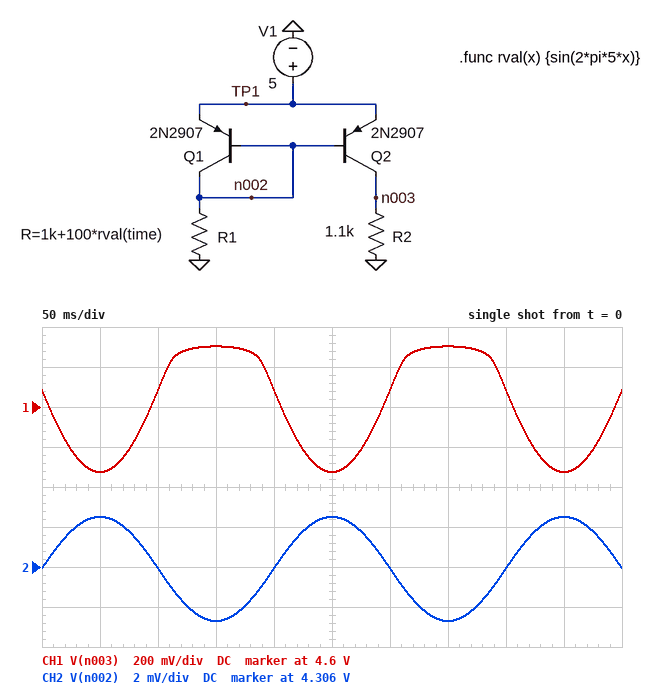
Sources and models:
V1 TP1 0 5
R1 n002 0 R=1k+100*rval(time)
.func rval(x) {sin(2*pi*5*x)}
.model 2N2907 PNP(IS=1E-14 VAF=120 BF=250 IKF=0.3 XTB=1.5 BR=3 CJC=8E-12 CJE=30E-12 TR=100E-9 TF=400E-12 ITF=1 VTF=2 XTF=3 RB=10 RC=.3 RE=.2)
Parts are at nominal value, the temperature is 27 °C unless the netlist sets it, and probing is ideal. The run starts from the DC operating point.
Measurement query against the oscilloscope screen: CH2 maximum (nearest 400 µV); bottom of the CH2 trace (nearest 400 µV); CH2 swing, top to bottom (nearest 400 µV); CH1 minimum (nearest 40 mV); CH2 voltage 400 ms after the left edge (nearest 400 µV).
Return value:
4.3084 V
4.3032 V
5.2 mV
4.28 V
4.3060 V
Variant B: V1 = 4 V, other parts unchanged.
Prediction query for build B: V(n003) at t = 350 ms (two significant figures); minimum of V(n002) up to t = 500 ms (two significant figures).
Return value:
3.9 V
3.3 V
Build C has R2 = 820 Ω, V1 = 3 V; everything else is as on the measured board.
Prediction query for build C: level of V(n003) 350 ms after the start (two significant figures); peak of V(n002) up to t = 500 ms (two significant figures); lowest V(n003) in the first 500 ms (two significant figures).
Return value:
2.1 V
2.3 V
1.7 V
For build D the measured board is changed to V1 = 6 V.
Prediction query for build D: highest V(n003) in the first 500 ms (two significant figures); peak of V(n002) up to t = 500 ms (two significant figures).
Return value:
5.9 V
5.3 V
